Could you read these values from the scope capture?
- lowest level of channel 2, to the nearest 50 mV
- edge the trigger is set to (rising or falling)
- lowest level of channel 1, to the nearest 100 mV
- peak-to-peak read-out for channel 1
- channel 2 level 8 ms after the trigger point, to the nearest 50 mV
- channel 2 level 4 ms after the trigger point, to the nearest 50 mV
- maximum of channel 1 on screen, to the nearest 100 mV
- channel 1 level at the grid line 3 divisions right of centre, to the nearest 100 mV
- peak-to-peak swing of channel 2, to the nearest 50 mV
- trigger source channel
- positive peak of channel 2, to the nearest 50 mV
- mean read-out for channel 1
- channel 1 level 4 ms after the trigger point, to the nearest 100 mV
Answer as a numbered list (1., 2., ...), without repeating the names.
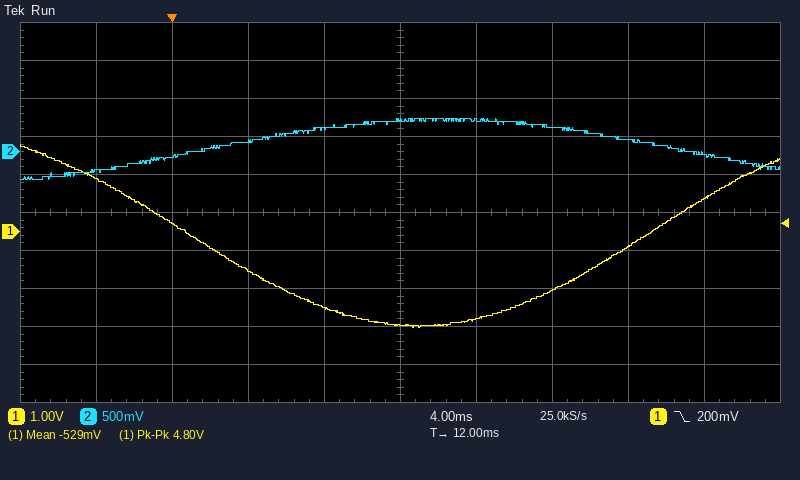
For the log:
1. -350 mV
2. falling
3. -2.5 V
4. 4.80 V
5. 300 mV
6. 150 mV
7. 2.3 V
8. -400 mV
9. 800 mV
10. channel 1
11. 450 mV
12. -529 mV
13. -1.0 V
